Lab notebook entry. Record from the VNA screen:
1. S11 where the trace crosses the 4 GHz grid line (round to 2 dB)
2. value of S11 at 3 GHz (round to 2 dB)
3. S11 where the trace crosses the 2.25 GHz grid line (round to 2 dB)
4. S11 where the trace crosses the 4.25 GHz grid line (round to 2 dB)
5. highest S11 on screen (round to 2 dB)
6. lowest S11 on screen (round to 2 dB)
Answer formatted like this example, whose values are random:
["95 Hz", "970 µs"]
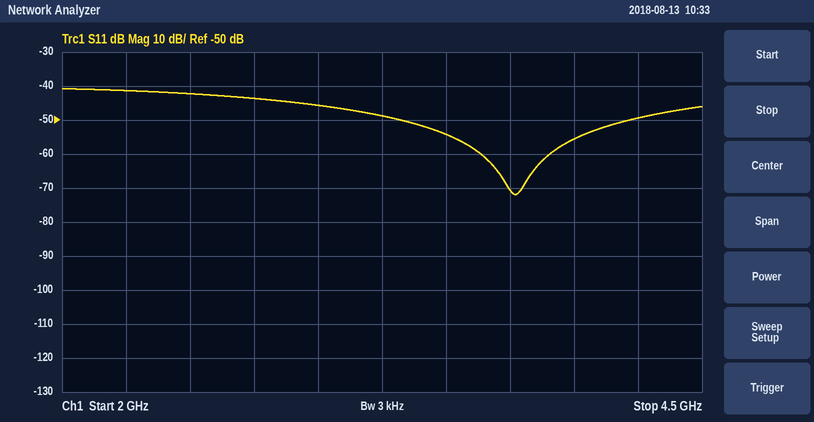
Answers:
["-56 dB", "-46 dB", "-42 dB", "-50 dB", "-40 dB", "-72 dB"]
